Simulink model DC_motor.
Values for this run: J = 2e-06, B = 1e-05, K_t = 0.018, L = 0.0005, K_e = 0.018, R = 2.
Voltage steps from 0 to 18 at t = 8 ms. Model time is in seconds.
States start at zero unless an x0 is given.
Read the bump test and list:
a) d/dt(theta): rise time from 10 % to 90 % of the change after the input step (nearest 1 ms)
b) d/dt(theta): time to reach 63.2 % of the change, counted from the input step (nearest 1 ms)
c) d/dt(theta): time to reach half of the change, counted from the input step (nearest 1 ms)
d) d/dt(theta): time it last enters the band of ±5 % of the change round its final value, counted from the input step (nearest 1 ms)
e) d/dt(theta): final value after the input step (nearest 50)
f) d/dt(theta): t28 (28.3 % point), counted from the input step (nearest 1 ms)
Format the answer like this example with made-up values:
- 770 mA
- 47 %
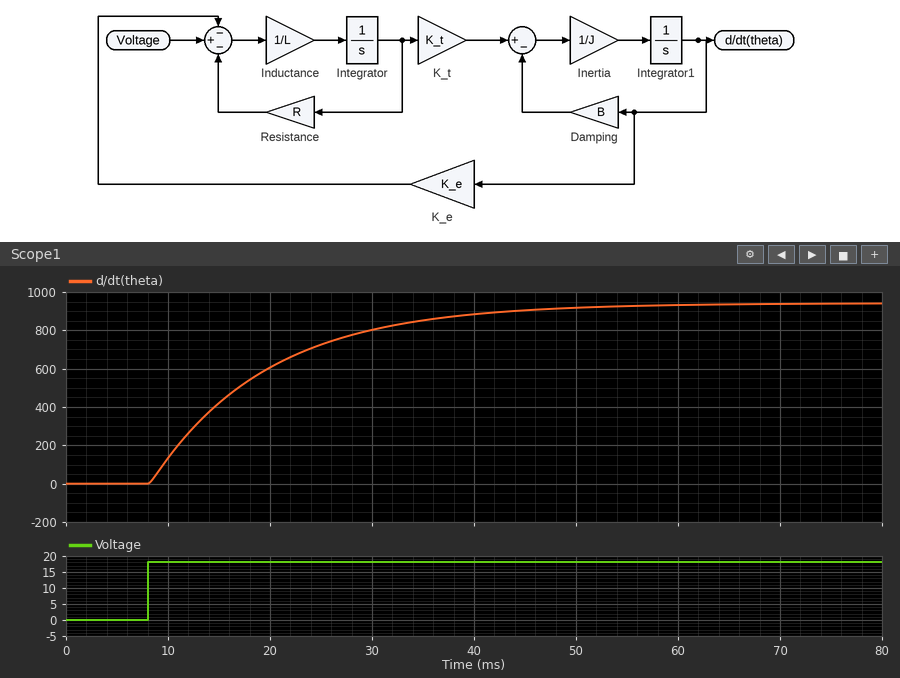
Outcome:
- 25 ms
- 12 ms
- 8 ms
- 34 ms
- 950
- 4 ms
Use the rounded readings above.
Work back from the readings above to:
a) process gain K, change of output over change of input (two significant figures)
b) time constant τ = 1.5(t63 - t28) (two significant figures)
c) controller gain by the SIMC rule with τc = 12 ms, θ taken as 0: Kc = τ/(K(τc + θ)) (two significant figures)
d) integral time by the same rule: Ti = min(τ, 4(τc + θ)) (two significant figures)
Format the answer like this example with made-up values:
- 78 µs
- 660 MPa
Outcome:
- 53
- 12 ms
- 0.019
- 12 ms
